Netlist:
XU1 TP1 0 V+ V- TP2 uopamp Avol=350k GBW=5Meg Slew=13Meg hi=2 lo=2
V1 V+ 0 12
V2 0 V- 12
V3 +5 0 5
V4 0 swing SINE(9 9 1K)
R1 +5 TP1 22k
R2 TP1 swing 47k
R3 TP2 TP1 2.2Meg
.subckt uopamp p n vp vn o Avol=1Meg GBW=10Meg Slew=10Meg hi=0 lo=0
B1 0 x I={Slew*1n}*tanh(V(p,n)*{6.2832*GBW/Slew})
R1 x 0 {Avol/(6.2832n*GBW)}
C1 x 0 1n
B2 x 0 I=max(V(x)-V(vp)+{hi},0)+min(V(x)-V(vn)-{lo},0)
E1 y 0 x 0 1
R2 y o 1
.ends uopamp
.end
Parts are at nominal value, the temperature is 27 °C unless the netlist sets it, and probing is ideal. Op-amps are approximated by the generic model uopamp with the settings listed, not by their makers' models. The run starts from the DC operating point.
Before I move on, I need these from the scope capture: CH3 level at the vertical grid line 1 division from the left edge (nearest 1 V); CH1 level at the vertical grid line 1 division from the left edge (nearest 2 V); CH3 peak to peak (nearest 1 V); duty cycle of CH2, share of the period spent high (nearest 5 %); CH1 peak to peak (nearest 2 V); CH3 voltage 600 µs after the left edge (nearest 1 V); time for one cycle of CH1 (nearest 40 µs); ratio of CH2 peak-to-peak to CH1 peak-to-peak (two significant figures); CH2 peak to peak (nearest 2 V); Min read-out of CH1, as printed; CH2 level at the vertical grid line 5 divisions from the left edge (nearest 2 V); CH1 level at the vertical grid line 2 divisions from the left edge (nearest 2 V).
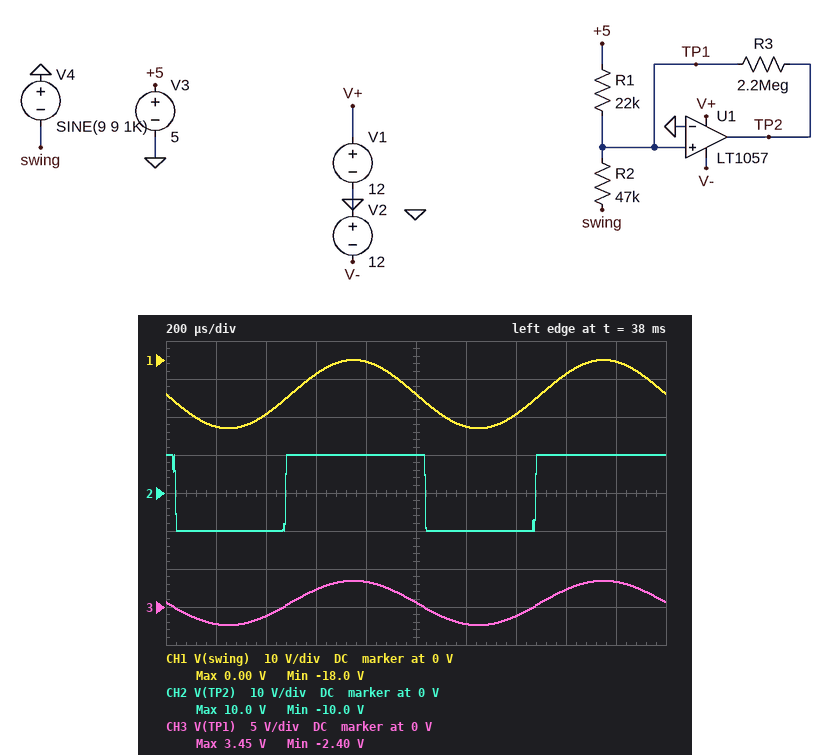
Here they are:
-2 V
-18 V
6 V
55 %
18 V
2 V
1.00 ms
1.1
20 V
-18.0 V
10 V
-14 V
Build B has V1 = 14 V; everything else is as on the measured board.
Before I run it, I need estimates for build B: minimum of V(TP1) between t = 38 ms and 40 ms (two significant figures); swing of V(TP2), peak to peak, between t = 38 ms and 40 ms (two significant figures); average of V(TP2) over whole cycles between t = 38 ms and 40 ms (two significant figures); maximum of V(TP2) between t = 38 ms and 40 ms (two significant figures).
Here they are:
-2.4 V
22 V
2.3 V
12 V
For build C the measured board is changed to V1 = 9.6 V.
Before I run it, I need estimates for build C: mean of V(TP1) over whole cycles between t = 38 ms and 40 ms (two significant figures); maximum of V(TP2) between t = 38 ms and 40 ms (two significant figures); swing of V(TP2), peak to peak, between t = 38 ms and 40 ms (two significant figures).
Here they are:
530 mV
7.6 V
18 V
